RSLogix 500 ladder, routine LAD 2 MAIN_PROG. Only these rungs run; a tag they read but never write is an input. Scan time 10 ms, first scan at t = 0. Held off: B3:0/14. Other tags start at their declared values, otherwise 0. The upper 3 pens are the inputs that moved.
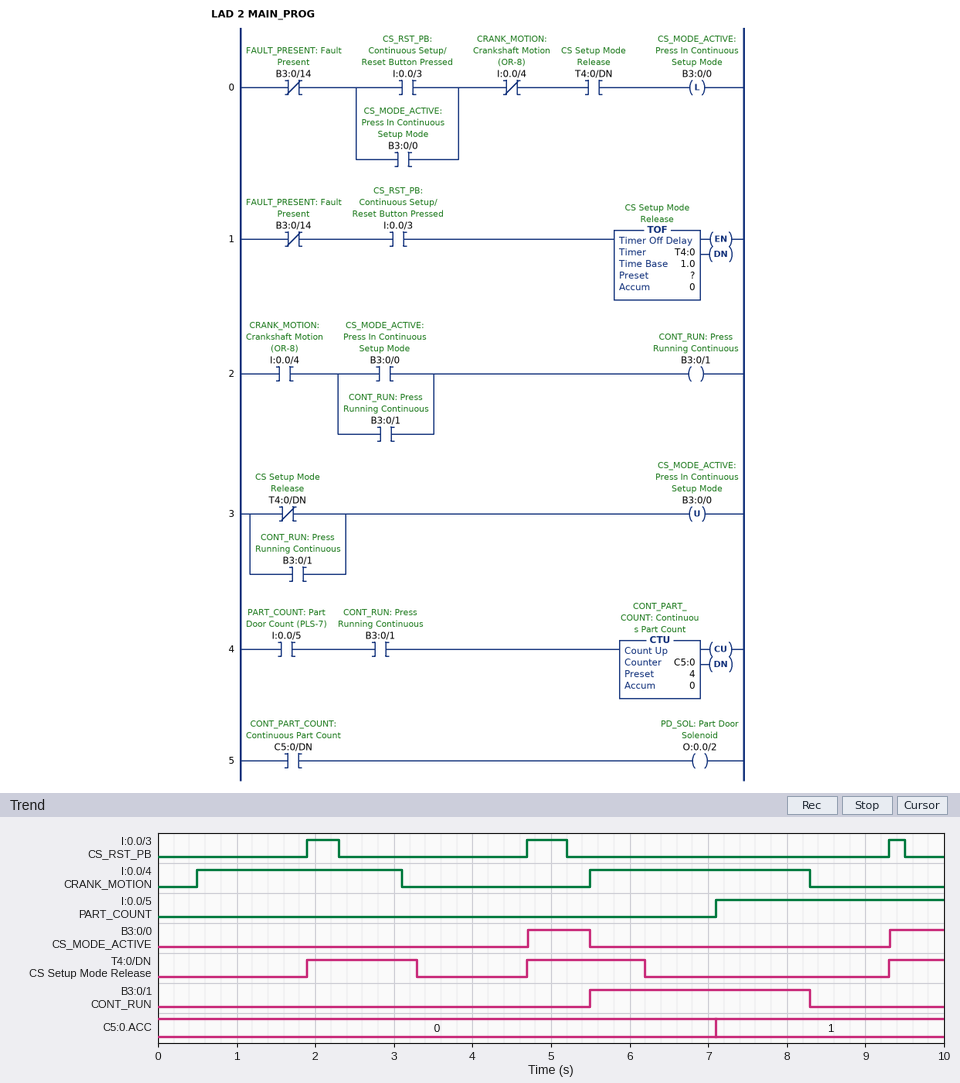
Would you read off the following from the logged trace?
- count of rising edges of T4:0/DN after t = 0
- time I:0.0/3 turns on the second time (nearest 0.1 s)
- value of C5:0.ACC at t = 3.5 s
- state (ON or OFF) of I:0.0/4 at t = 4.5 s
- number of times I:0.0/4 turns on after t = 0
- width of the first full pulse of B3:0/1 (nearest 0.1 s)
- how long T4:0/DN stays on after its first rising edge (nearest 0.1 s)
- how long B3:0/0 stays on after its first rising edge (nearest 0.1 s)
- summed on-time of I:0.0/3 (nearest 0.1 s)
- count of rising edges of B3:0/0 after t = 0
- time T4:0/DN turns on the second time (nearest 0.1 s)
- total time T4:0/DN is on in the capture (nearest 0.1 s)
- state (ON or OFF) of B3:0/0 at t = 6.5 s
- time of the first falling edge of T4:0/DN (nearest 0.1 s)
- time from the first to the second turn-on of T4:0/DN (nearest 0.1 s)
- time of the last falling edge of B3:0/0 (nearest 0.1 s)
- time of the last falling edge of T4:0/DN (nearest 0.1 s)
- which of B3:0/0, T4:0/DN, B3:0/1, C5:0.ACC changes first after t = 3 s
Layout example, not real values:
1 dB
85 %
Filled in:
3
4.7 s
0
OFF
2
2.8 s
1.4 s
0.8 s
1.1 s
2
4.7 s
3.6 s
OFF
3.3 s
2.8 s
5.5 s
6.2 s
T4:0/DN
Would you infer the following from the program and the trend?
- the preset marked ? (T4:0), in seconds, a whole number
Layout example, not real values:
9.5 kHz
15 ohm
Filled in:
1 s
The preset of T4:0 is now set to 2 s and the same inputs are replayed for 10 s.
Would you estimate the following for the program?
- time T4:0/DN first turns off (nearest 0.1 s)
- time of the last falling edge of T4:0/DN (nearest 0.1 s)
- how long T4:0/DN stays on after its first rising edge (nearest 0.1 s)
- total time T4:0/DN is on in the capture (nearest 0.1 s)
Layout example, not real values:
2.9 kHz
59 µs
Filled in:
4.3 s
7.2 s
2.4 s
5.6 s
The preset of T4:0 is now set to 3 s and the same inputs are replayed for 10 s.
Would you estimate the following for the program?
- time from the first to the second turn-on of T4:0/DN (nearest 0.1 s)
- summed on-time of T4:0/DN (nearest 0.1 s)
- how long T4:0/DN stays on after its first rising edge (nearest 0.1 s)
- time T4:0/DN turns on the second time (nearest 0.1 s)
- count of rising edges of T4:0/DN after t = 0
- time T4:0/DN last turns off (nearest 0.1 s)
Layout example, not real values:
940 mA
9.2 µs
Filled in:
7.4 s
7.0 s
6.3 s
9.3 s
2
8.2 s
